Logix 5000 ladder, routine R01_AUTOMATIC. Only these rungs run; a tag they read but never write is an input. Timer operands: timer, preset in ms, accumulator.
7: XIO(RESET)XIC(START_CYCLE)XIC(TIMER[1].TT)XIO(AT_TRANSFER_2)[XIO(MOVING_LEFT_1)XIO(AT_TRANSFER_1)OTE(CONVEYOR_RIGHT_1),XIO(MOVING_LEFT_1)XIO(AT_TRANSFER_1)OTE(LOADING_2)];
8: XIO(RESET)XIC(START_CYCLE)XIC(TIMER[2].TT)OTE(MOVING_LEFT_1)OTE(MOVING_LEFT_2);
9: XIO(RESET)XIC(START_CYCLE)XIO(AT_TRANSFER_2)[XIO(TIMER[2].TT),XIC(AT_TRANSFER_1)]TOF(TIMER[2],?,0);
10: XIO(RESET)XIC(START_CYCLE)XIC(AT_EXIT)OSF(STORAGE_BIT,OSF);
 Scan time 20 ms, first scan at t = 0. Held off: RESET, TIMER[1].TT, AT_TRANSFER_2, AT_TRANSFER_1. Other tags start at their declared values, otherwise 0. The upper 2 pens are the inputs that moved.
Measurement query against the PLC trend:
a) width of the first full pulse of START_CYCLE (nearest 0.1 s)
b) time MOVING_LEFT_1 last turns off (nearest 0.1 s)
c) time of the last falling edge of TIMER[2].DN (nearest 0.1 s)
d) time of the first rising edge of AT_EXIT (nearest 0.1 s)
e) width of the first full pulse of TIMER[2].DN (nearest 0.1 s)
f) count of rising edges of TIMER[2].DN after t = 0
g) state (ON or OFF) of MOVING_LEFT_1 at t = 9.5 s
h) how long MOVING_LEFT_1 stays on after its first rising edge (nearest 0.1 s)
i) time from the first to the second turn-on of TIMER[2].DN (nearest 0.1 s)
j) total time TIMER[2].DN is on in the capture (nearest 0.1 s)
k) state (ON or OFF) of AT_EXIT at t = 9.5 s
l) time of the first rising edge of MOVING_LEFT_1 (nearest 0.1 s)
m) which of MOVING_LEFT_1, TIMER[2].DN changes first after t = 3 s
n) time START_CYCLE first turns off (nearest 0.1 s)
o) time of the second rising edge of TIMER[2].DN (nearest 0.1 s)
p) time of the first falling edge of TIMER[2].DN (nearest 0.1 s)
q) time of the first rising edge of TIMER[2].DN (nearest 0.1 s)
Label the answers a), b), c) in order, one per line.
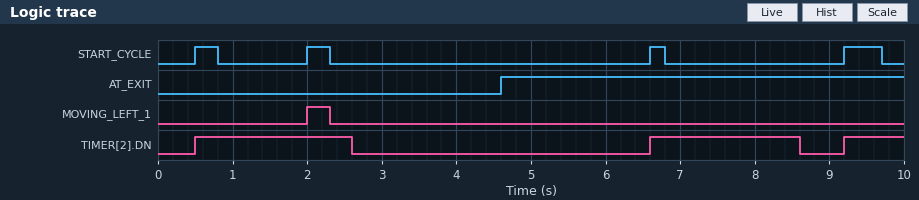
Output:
a) 0.3 s
b) 2.3 s
c) 8.6 s
d) 4.6 s
e) 2.1 s
f) 3
g) OFF
h) 0.3 s
i) 6.1 s
j) 4.9 s
k) ON
l) 2.0 s
m) TIMER[2].DN
n) 0.8 s
o) 6.6 s
p) 2.6 s
q) 0.5 s
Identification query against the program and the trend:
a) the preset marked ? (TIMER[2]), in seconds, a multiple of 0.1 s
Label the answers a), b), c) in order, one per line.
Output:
a) 1.8 s
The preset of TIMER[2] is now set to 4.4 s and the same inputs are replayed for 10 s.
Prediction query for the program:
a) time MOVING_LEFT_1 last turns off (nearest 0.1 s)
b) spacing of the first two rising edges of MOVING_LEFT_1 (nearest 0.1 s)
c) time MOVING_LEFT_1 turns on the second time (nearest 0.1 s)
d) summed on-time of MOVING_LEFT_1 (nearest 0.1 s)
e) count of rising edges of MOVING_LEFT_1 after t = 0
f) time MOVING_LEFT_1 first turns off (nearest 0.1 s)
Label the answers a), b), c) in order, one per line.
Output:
a) 9.7 s
b) 7.2 s
c) 9.2 s
d) 0.8 s
e) 2
f) 2.3 s
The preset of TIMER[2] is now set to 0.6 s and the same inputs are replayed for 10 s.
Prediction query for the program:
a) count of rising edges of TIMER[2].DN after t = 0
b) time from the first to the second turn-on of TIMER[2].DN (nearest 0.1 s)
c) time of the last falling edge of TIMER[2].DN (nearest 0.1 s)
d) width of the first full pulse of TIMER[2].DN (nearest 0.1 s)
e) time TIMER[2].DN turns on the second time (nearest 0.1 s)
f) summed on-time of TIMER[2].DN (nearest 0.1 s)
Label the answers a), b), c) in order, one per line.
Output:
a) 4
b) 1.5 s
c) 7.4 s
d) 0.9 s
e) 2.0 s
f) 3.4 s
